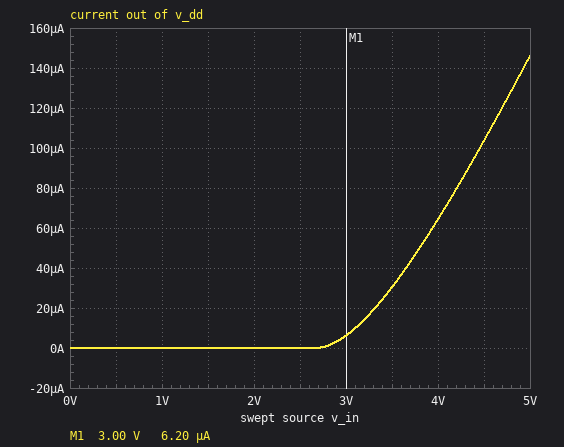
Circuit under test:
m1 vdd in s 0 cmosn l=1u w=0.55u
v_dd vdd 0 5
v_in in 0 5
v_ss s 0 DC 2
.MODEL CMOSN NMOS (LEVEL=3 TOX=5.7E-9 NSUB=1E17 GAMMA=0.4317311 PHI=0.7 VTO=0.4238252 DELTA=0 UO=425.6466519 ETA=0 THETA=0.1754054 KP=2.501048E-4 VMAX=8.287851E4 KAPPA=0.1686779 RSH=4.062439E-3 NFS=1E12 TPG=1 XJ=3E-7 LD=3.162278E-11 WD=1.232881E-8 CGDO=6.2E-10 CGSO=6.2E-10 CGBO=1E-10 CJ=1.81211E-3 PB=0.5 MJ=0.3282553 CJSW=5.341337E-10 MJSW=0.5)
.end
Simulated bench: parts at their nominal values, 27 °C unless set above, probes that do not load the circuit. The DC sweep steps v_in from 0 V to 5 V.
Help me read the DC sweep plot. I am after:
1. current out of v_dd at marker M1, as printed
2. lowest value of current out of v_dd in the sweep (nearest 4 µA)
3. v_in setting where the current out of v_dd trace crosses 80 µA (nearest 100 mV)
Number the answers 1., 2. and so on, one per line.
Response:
1. 6.20 µA
2. 0 A
3. 4.2 V
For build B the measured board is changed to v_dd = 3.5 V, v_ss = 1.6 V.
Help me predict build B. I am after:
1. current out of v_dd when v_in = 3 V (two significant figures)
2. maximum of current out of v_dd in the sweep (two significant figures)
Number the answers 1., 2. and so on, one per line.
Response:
1. 26 µA
2. 180 µA
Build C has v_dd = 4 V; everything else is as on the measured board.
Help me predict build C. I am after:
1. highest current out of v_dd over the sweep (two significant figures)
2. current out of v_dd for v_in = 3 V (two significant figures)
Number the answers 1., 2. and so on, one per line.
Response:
1. 140 µA
2. 6.1 µA
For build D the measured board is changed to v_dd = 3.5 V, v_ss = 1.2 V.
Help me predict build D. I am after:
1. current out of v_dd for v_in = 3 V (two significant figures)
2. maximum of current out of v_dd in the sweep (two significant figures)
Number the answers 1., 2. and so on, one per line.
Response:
1. 55 µA
2. 220 µA
